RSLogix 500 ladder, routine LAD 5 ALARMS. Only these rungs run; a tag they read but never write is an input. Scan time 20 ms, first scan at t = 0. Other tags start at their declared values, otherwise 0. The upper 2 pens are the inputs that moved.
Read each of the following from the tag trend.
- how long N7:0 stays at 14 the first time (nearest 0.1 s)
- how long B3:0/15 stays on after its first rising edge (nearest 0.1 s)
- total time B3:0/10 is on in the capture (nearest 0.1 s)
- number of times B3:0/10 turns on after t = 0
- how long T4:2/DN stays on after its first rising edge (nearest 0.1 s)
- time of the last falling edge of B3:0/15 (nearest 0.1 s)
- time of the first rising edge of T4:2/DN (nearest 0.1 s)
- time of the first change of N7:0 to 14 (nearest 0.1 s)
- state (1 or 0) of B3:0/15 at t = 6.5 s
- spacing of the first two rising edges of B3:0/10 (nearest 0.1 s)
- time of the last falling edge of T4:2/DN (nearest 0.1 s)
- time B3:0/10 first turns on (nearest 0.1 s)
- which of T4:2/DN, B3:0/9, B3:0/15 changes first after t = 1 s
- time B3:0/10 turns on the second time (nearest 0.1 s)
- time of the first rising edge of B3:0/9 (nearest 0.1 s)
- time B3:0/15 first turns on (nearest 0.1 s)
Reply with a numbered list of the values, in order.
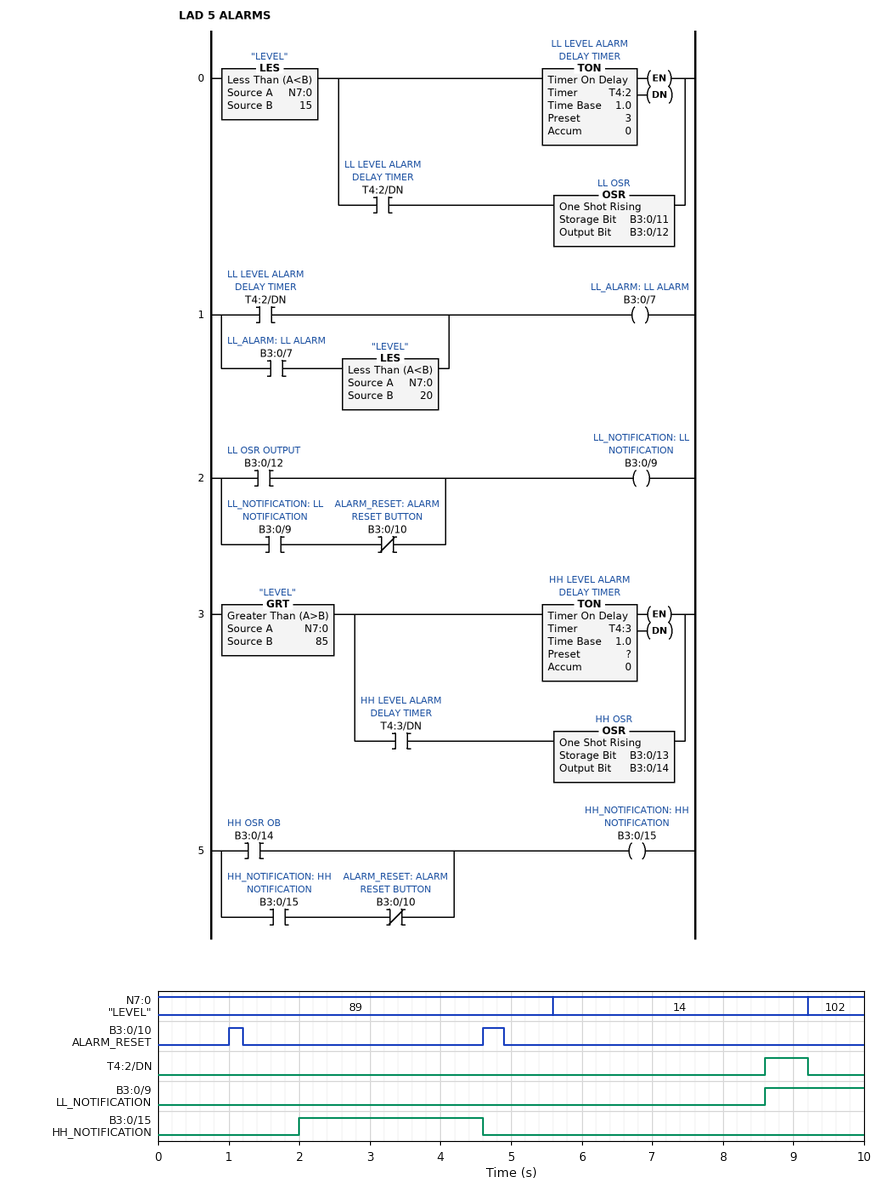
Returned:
1. 3.6 s
2. 2.6 s
3. 0.5 s
4. 2
5. 0.6 s
6. 4.6 s
7. 8.6 s
8. 5.6 s
9. 0
10. 3.6 s
11. 9.2 s
12. 1.0 s
13. B3:0/15
14. 4.6 s
15. 8.6 s
16. 2.0 s
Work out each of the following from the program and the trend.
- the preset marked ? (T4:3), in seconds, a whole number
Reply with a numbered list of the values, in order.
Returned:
1. 2 s
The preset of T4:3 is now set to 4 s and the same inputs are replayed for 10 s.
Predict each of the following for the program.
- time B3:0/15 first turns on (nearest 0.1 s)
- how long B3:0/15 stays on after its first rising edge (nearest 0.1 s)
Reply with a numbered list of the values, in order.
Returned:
1. 4.0 s
2. 0.6 s
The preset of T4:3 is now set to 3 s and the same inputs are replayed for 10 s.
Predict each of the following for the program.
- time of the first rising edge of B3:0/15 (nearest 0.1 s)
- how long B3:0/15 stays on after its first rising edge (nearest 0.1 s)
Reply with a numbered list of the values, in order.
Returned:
1. 3.0 s
2. 1.6 s
